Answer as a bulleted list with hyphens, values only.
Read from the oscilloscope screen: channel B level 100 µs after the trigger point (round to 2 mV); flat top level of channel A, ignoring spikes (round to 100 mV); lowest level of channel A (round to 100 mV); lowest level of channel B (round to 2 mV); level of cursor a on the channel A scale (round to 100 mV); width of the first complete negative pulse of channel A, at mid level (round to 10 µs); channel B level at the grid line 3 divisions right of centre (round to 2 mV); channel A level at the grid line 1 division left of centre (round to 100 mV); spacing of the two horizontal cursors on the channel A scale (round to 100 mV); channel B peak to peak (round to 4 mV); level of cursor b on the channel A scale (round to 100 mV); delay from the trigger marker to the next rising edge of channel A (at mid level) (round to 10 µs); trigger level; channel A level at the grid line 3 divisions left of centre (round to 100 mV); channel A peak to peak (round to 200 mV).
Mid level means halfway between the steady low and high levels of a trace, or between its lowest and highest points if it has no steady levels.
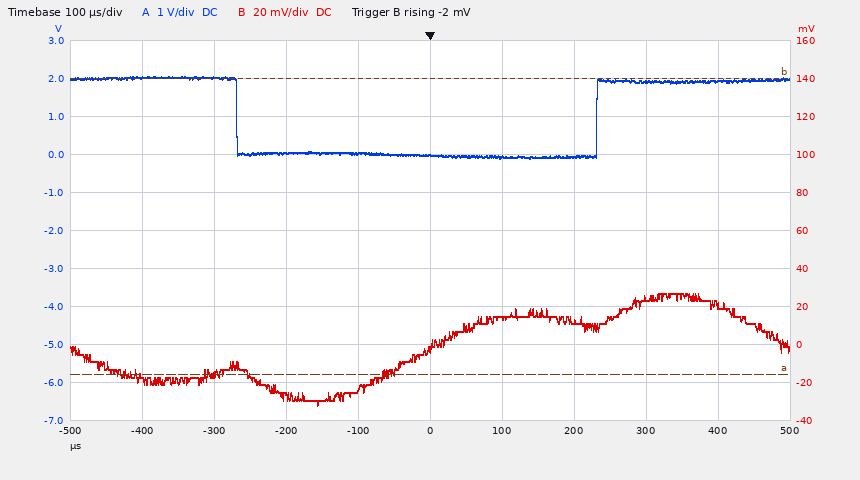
- 14 mV
- 2.0 V
- -100 mV
- -32 mV
- -5.8 V
- 500 µs
- 24 mV
- 0.0 V
- 7.8 V
- 60 mV
- 2.0 V
- 230 µs
- -2 mV
- 2.0 V
- 2.2 V
